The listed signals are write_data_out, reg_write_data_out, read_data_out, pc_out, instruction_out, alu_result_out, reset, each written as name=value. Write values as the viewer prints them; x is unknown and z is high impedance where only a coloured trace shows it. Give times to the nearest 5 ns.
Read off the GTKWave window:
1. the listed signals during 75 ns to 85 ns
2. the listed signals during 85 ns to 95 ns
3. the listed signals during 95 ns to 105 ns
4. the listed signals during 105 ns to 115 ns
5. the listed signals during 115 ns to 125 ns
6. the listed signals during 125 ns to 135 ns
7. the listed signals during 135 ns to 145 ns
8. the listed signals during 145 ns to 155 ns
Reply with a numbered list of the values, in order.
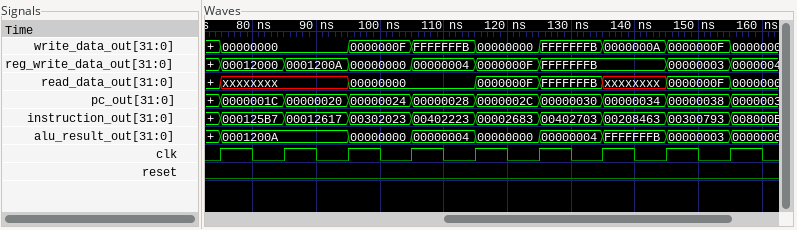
1. write_data_out=00000000, reg_write_data_out=00012000, read_data_out=xxxxxxxx, pc_out=0000001C, instruction_out=000125B7, alu_result_out=0001200A, reset=0
2. write_data_out=00000000, reg_write_data_out=0001200A, read_data_out=xxxxxxxx, pc_out=00000020, instruction_out=00012617, alu_result_out=0001200A, reset=0
3. write_data_out=0000000F, reg_write_data_out=00000000, read_data_out=00000000, pc_out=00000024, instruction_out=00302023, alu_result_out=00000000, reset=0
4. write_data_out=FFFFFFFB, reg_write_data_out=00000004, read_data_out=00000000, pc_out=00000028, instruction_out=00402223, alu_result_out=00000004, reset=0
5. write_data_out=00000000, reg_write_data_out=0000000F, read_data_out=0000000F, pc_out=0000002C, instruction_out=00002683, alu_result_out=00000000, reset=0
6. write_data_out=FFFFFFFB, reg_write_data_out=FFFFFFFB, read_data_out=FFFFFFFB, pc_out=00000030, instruction_out=00402703, alu_result_out=00000004, reset=0
7. write_data_out=0000000A, reg_write_data_out=FFFFFFFB, read_data_out=xxxxxxxx, pc_out=00000034, instruction_out=00208463, alu_result_out=FFFFFFFB, reset=0
8. write_data_out=0000000F, reg_write_data_out=00000003, read_data_out=0000000F, pc_out=00000038, instruction_out=00300793, alu_result_out=00000003, reset=0
